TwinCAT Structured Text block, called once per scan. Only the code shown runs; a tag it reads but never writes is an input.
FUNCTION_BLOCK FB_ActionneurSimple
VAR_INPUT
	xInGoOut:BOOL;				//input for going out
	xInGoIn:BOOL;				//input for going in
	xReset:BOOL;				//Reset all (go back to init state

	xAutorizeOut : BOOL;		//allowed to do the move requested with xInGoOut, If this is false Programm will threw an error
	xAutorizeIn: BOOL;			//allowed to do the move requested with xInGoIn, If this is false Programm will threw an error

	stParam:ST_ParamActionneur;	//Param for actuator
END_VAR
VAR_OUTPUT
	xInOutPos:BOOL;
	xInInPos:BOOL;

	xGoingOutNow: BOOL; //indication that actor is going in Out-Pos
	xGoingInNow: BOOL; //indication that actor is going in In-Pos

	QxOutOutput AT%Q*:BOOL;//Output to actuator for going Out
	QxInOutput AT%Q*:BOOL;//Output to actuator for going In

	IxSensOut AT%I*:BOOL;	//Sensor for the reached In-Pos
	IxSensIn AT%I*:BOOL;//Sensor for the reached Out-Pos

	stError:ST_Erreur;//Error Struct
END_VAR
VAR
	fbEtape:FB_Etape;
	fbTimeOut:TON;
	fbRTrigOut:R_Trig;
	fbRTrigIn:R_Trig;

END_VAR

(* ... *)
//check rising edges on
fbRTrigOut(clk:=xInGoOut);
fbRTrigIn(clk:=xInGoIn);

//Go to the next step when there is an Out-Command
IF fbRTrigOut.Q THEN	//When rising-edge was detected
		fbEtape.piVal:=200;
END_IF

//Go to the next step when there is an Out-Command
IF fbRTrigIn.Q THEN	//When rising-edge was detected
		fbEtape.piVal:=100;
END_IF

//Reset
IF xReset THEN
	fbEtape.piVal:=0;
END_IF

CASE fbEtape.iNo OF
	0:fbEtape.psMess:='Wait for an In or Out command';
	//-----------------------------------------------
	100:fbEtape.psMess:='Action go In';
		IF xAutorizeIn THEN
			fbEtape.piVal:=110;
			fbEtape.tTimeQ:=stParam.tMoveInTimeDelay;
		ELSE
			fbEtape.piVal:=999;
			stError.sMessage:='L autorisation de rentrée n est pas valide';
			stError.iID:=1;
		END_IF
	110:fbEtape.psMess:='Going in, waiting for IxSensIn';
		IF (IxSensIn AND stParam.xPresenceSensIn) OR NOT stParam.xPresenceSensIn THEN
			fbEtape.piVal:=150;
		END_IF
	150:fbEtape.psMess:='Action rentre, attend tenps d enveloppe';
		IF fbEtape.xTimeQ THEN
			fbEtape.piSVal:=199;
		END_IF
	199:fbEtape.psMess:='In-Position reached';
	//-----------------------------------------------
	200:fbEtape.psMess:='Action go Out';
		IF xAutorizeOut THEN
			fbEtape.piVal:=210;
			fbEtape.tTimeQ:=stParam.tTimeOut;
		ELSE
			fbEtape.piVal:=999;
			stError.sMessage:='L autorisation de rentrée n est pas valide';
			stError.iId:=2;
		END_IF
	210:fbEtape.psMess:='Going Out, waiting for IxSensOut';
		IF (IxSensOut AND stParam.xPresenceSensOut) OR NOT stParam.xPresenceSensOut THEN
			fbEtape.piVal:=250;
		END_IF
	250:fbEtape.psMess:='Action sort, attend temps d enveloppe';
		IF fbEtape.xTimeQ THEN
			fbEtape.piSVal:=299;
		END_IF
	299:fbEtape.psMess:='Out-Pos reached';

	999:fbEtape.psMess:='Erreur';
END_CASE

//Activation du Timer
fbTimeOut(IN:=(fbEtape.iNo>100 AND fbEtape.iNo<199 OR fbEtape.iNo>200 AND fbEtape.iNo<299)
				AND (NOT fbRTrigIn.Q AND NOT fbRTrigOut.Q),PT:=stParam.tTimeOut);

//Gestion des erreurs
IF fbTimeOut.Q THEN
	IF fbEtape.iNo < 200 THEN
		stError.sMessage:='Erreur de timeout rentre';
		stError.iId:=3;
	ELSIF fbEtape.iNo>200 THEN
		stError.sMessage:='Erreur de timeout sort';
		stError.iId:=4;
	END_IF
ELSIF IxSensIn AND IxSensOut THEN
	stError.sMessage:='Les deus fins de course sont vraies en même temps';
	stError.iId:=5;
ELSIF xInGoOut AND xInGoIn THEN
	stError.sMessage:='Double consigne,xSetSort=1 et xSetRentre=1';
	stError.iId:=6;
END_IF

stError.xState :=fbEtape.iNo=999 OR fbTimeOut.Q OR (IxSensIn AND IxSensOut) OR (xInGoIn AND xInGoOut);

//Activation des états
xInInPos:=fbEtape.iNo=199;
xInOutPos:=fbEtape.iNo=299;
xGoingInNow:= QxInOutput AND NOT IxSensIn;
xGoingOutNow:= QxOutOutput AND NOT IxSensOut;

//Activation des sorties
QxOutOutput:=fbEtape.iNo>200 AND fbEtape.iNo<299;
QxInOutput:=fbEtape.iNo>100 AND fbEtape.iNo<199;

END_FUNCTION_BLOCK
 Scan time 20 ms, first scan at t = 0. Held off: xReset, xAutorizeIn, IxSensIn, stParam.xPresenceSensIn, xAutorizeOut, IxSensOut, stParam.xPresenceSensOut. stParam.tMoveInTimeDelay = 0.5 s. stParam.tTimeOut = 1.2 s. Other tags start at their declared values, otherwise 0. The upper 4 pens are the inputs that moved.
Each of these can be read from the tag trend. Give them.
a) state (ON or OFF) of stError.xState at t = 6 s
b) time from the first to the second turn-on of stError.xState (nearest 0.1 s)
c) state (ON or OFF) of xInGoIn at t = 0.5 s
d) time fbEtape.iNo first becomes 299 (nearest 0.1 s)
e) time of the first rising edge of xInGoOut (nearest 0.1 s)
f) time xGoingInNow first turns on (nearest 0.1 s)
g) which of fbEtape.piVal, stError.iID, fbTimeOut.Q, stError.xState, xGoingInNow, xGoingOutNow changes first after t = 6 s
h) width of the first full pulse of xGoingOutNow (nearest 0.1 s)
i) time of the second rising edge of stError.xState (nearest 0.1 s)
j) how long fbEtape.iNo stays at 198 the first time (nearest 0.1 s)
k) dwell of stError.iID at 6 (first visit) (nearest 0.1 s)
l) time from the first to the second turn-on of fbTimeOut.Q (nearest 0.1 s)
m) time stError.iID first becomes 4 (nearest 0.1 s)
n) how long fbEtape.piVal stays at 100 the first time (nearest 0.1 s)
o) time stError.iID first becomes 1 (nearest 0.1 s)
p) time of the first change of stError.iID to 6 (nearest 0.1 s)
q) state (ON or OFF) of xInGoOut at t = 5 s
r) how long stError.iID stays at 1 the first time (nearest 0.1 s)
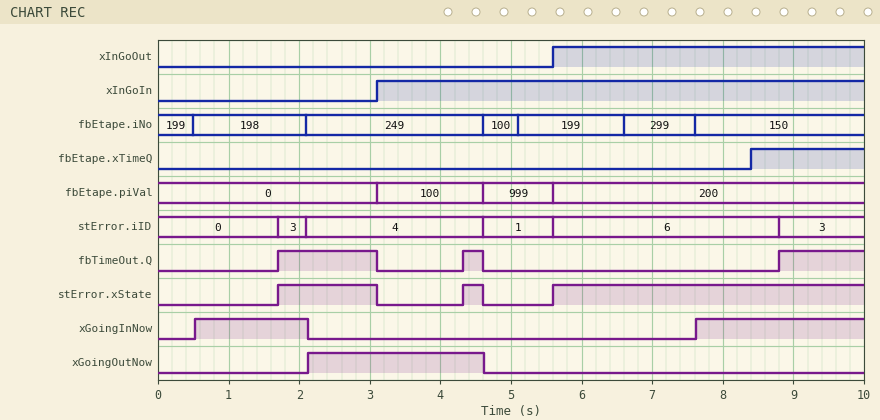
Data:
ON
2.6 s
OFF
6.6 s
5.6 s
0.5 s
xGoingInNow
2.5 s
4.3 s
1.6 s
3.2 s
2.6 s
2.1 s
1.5 s
4.6 s
5.6 s
OFF
1.0 s
